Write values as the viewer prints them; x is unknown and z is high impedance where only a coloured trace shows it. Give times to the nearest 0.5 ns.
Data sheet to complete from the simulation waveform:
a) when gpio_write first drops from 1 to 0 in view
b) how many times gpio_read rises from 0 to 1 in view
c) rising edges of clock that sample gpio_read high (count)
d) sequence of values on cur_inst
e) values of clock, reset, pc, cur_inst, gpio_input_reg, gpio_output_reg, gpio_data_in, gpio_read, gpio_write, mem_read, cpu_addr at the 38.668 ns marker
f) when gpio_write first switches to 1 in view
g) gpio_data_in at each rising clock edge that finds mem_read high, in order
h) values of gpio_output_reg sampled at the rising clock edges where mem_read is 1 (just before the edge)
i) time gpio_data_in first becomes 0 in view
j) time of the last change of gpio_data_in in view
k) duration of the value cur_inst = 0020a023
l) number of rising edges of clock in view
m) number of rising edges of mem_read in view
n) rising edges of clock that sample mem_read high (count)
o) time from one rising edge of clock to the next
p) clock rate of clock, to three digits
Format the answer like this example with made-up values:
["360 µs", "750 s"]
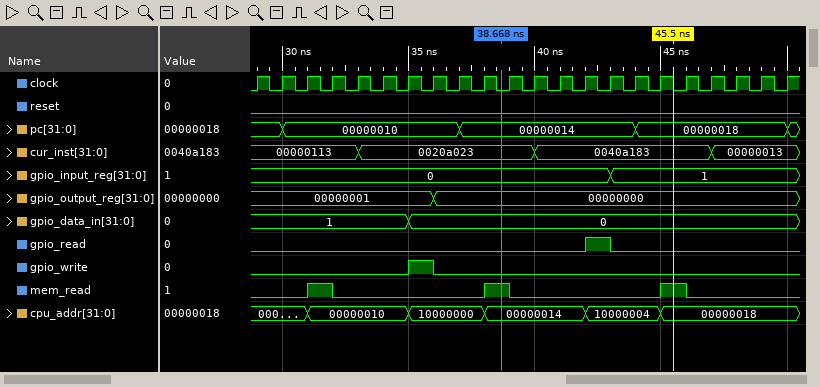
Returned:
["36 ns", "1", "1", "00000113, 0020a023, 0040a183, 00000013", "clock=0, reset=0, pc=00000014, cur_inst=0020a023, gpio_input_reg=0, gpio_output_reg=00000000, gpio_data_in=0, gpio_read=0, gpio_write=0, mem_read=1, cpu_addr=00000014", "35 ns", "1, 0, 0", "00000001, 00000000, 00000000", "35 ns", "35 ns", "7 ns", "22", "3", "3", "1 ns", "1.00 GHz"]
